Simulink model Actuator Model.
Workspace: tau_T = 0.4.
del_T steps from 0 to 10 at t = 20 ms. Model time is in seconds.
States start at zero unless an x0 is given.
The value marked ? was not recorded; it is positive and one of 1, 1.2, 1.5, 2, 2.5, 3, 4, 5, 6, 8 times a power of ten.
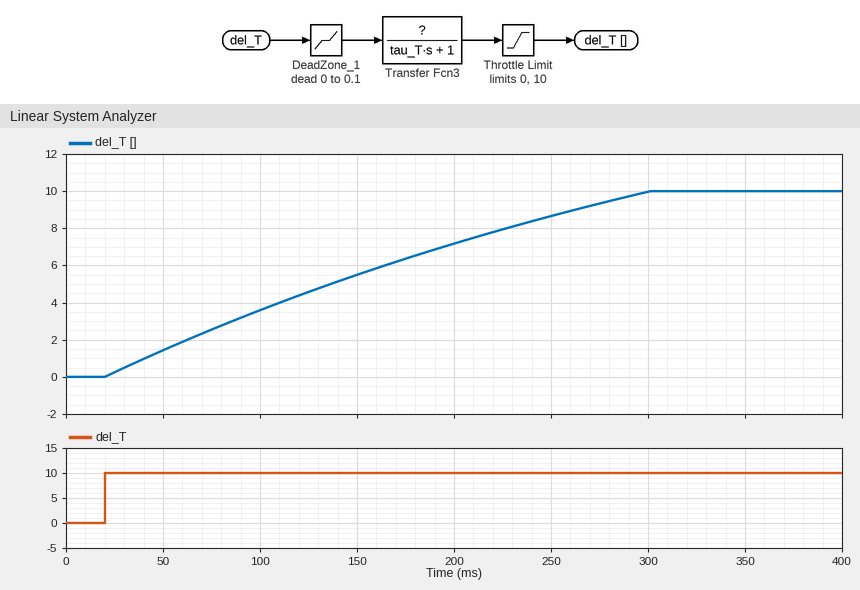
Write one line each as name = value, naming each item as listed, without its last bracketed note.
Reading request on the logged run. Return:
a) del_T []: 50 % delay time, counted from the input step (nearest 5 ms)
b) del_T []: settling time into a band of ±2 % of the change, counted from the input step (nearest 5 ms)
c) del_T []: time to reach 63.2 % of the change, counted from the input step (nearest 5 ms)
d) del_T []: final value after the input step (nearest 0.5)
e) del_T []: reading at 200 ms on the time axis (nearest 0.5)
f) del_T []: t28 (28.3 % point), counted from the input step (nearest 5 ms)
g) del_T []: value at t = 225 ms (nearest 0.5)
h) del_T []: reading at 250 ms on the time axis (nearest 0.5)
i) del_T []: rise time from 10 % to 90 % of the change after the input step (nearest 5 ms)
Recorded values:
del_T []: 50 % delay time, counted from the input step = 115 ms
del_T []: settling time into a band of ±2 % of the change, counted from the input step = 275 ms
del_T []: time to reach 63.2 % of the change, counted from the input step = 155 ms
del_T []: final value after the input step = 10.0
del_T []: reading at 200 ms on the time axis = 7.0
del_T []: t28 (28.3 % point), counted from the input step = 60 ms
del_T []: value at t = 225 ms = 8.0
del_T []: reading at 250 ms on the time axis = 8.5
del_T []: rise time from 10 % to 90 % of the change after the input step = 220 ms
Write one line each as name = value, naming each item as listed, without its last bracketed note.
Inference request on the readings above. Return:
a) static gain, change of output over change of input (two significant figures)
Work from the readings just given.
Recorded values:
static gain, change of output over change of input = 1.0
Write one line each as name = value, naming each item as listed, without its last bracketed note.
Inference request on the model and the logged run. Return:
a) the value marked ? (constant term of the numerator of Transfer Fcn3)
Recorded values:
the value marked ? = 2
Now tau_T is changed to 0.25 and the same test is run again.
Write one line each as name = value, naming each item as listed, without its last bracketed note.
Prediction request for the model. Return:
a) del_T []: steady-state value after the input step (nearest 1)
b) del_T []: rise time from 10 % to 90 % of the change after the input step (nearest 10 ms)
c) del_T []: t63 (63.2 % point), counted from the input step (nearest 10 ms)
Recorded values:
del_T []: steady-state value after the input step = 10
del_T []: rise time from 10 % to 90 % of the change after the input step = 140 ms
del_T []: t63 (63.2 % point), counted from the input step = 100 ms
